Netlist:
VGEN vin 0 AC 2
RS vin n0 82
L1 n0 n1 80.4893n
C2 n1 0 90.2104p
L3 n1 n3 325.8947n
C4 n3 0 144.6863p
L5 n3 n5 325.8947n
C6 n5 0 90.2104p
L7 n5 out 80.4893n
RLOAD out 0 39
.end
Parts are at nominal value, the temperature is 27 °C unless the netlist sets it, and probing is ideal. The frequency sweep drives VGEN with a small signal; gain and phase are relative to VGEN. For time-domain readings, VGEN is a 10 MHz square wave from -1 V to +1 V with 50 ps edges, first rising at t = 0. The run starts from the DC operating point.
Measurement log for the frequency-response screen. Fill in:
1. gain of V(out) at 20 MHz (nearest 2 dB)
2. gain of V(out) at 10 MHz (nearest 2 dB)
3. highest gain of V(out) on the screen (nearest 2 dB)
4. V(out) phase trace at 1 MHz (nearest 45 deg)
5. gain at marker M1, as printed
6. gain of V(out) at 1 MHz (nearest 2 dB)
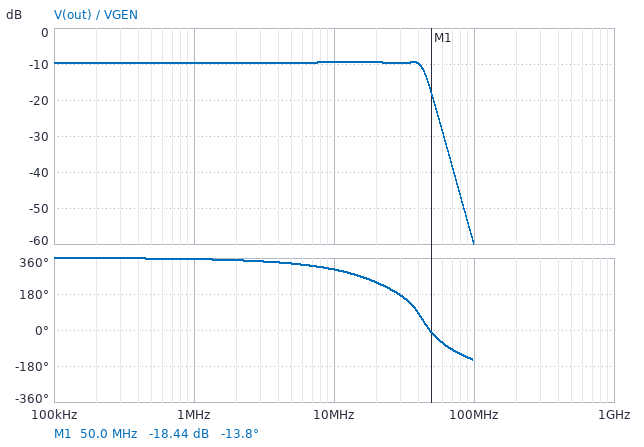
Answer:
-10 dB
-10 dB
-10 dB
360 deg
-18.44 dB
-10 dB
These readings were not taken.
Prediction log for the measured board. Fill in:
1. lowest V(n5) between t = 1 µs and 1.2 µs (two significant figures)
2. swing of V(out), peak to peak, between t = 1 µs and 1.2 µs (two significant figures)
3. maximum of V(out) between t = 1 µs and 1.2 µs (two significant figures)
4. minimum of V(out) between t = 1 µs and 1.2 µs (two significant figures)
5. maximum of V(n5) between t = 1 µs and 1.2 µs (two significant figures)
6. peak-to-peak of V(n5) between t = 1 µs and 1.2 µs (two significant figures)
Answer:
-460 mV
880 mV
440 mV
-440 mV
460 mV
920 mV
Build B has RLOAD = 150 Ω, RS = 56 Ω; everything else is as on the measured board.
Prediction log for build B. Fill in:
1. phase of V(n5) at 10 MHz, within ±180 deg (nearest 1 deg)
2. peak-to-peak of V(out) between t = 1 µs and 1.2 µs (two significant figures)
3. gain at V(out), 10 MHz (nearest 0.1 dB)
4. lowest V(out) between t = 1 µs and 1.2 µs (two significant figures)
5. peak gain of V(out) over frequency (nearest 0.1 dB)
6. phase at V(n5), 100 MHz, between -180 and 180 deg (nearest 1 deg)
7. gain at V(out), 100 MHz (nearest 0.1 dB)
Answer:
-58 deg
1.8 V
-3.1 dB
-910 mV
-1.8 dB
-112 deg
-55.4 dB
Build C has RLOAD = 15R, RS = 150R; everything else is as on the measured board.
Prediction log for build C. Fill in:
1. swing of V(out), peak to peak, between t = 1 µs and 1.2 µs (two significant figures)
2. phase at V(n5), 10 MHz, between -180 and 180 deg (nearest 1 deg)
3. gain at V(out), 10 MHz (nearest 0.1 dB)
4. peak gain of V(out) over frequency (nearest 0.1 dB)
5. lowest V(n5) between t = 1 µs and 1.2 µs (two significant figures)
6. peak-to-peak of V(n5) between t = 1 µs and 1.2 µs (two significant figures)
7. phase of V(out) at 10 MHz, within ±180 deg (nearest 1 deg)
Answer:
350 mV
-25 deg
-17.9 dB
-16.0 dB
-210 mV
430 mV
-44 deg
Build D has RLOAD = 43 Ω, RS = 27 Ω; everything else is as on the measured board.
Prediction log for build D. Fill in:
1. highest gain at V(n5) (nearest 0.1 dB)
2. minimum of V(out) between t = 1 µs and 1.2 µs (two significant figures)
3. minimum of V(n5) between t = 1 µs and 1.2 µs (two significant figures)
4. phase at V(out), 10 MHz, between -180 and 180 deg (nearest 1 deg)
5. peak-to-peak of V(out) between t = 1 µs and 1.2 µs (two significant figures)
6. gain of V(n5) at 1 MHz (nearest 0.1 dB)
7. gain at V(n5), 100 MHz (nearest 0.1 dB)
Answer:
-3.8 dB
-750 mV
-780 mV
-60 deg
1.5 V
-4.2 dB
-49.5 dB
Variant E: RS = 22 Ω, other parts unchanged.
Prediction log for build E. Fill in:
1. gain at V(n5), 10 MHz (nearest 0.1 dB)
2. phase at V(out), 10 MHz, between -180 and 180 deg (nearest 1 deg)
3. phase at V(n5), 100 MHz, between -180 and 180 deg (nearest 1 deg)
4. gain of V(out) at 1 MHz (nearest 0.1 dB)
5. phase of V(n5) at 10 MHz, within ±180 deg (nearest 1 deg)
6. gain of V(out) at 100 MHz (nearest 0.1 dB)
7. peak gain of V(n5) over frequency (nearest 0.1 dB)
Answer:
-4.4 dB
-61 deg
-131 deg
-3.9 dB
-54 deg
-52.9 dB
-3.3 dB
